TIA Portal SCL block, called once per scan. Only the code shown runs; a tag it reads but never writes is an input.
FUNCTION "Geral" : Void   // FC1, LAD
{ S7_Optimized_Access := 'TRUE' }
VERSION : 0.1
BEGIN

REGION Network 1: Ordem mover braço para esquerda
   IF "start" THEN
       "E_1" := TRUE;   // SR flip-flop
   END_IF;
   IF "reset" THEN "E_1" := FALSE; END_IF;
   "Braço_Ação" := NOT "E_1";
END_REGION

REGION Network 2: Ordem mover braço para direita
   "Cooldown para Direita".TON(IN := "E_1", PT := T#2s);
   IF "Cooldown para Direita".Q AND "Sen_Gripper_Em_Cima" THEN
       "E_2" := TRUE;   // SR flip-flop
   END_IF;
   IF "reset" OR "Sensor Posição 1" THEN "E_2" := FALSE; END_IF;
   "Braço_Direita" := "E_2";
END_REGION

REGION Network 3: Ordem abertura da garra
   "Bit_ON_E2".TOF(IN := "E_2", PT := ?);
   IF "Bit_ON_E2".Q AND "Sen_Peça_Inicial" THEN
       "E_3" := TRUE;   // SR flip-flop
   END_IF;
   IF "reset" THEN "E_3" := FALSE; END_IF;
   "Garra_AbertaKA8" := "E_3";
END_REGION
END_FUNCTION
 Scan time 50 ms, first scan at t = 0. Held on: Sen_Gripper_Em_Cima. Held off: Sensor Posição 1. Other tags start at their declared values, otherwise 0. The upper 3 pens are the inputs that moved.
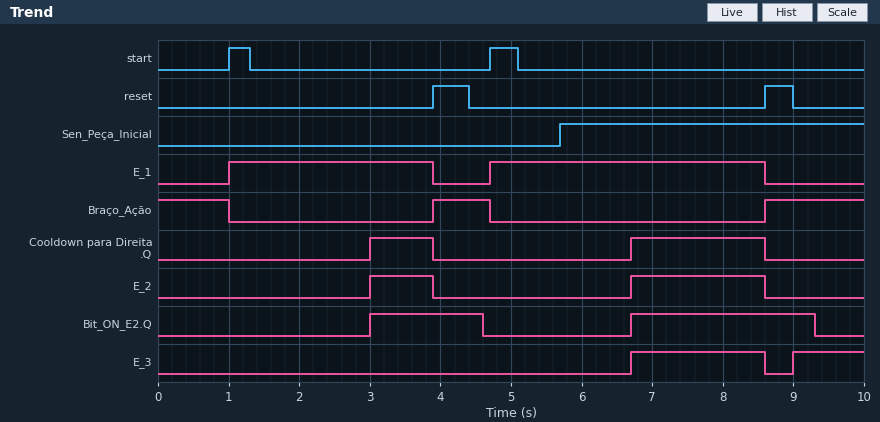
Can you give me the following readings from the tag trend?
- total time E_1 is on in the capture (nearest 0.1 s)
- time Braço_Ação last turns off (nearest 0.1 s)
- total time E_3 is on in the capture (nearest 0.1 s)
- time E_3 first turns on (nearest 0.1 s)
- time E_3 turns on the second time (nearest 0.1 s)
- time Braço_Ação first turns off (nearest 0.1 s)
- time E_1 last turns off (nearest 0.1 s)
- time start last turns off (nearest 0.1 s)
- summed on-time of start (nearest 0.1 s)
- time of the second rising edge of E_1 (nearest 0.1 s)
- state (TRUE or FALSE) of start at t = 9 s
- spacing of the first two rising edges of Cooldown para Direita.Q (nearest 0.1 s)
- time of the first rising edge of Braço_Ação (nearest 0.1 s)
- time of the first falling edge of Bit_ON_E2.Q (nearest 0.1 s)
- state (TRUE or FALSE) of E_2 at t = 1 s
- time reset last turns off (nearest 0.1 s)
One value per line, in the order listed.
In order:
6.8 s
4.7 s
2.9 s
6.7 s
9.0 s
1.0 s
8.6 s
5.1 s
0.7 s
4.7 s
FALSE
3.7 s
3.9 s
4.6 s
FALSE
9.0 s
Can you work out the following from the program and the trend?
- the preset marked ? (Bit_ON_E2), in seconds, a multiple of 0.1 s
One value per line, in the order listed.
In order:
0.7 s
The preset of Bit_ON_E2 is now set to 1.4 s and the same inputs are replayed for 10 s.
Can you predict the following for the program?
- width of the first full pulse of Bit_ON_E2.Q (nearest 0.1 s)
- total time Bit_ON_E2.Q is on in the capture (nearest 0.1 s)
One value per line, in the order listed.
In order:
2.3 s
5.6 s
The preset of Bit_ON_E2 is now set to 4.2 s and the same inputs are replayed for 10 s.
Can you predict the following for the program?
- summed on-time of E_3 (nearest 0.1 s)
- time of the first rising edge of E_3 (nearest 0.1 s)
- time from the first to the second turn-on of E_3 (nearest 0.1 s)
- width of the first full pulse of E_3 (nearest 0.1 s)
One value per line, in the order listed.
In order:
3.9 s
5.7 s
3.3 s
2.9 s
